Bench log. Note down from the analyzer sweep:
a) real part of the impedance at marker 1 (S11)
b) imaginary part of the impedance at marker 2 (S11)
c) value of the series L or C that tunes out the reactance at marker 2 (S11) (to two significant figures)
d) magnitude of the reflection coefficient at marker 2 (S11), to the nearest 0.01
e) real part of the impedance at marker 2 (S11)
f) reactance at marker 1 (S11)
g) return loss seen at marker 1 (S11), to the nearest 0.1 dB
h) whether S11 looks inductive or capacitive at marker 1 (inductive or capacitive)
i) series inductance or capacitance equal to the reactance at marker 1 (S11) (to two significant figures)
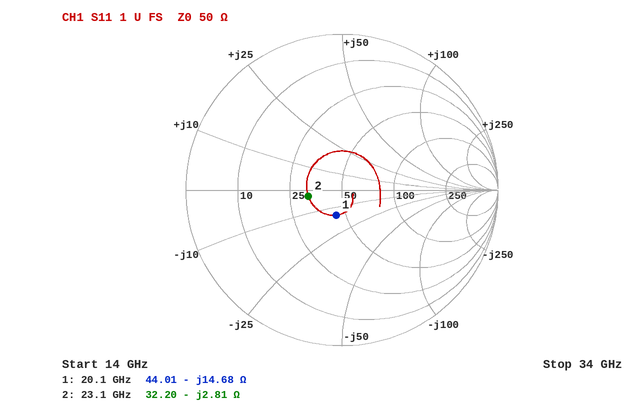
44.01 Ω
-2.81 Ω
19 pH
0.22
32.20 Ω
-14.68 Ω
15.6 dB
capacitive
540 fF
